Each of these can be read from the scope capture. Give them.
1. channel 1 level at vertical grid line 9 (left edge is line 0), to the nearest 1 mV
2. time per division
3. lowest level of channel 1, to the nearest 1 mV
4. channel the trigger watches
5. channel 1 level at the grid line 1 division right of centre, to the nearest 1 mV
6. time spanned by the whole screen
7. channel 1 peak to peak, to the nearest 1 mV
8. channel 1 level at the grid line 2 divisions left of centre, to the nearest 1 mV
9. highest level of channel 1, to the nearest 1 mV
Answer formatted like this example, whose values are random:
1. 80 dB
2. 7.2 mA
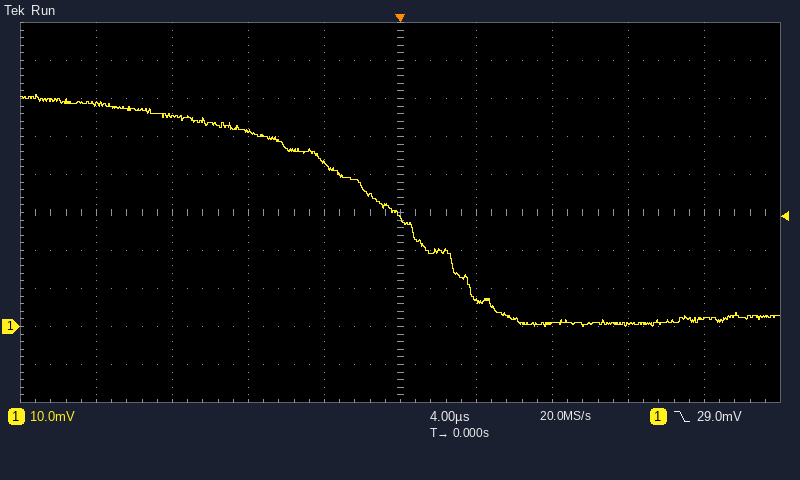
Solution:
1. 2 mV
2. 4 µs
3. 0 mV
4. channel 1
5. 7 mV
6. 40 µs
7. 61 mV
8. 51 mV
9. 61 mV
